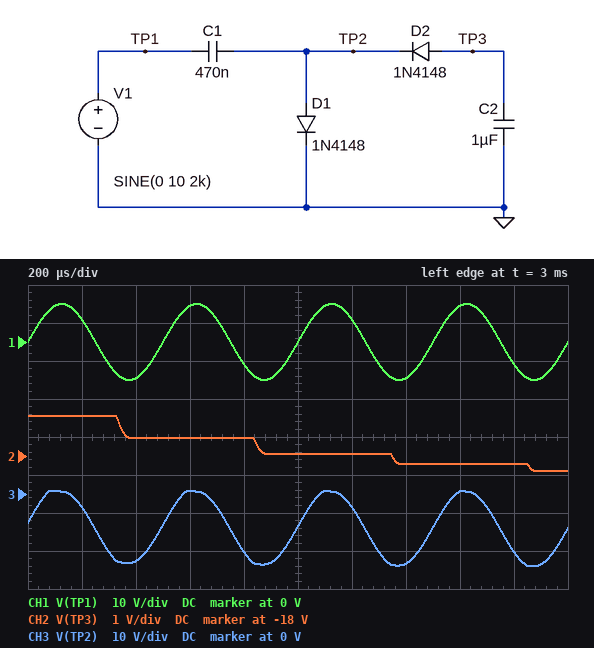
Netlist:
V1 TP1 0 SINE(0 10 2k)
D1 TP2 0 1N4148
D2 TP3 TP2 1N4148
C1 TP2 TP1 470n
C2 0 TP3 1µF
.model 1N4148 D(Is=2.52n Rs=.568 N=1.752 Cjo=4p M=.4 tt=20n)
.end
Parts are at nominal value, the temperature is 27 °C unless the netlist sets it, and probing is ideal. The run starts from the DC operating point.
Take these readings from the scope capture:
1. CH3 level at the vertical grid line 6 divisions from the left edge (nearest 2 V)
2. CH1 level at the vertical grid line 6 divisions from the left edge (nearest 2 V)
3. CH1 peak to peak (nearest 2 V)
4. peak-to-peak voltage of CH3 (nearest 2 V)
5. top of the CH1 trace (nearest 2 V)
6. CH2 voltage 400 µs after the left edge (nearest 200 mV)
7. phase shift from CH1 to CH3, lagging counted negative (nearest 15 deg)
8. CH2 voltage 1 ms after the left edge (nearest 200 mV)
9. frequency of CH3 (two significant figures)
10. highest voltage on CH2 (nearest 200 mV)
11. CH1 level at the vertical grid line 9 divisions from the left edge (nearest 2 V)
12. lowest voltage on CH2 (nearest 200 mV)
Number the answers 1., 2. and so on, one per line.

1. -4 V
2. 6 V
3. 20 V
4. 20 V
5. 10 V
6. -17.6 V
7. 0 deg
8. -18.0 V
9. 2.0 kHz
10. -17.0 V
11. -6 V
12. -18.4 V
